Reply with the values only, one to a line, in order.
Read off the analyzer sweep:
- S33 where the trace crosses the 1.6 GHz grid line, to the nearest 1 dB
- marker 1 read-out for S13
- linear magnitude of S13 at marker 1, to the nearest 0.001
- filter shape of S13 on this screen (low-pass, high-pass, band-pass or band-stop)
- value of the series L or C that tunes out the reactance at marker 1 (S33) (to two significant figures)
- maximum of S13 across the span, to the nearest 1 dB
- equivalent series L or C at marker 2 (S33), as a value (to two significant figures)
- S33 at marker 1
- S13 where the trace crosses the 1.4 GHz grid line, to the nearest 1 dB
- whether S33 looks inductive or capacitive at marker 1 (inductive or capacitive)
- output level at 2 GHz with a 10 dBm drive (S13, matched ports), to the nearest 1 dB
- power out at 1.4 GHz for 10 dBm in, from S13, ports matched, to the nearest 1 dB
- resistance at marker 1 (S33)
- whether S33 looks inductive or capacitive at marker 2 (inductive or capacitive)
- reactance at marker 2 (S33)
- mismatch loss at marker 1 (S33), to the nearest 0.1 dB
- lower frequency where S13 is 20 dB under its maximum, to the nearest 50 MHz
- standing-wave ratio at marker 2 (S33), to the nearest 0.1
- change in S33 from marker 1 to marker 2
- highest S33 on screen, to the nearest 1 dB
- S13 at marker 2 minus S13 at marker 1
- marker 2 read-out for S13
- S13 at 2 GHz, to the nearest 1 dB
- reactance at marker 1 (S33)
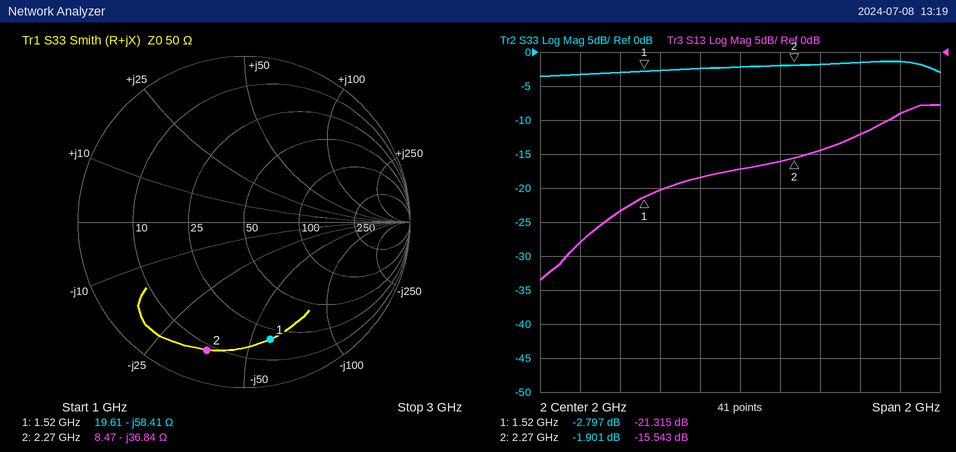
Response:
-3 dB
-21.315 dB
0.086
high-pass
6.1 nH
-8 dB
1.9 pF
-2.797 dB
-23 dB
capacitive
-7 dBm
-13 dBm
19.61 Ω
capacitive
-36.84 Ω
3.2 dB
1.20 GHz
9.2
0.896 dB
-1 dB
5.772 dB
-15.543 dB
-17 dB
-58.41 Ω
